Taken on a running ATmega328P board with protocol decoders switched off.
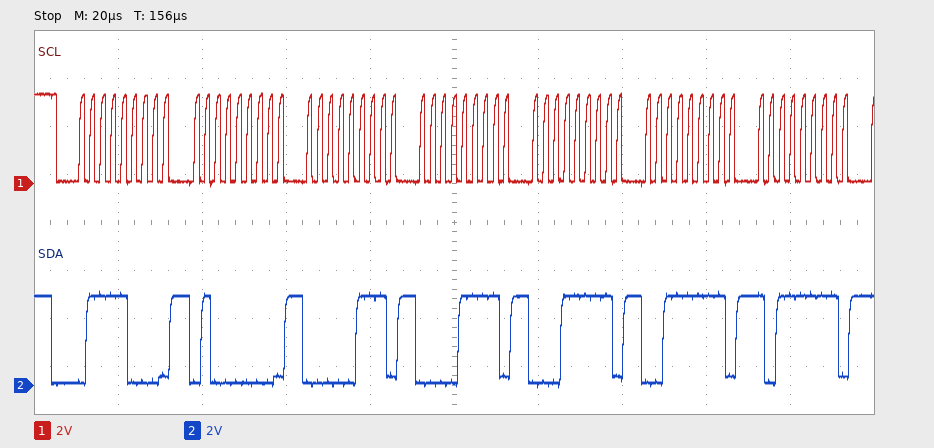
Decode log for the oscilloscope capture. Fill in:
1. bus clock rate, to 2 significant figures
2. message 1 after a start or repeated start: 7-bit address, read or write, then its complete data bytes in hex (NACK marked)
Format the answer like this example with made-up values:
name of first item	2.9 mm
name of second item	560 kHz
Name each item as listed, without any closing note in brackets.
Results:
bus clock rate, to 2 significant figures	400 kHz
message 1 after a start or repeated start: 7-bit address, read or write, then its complete data bytes in hex	0x3C write: 40 07 0F 1F 3F BF
